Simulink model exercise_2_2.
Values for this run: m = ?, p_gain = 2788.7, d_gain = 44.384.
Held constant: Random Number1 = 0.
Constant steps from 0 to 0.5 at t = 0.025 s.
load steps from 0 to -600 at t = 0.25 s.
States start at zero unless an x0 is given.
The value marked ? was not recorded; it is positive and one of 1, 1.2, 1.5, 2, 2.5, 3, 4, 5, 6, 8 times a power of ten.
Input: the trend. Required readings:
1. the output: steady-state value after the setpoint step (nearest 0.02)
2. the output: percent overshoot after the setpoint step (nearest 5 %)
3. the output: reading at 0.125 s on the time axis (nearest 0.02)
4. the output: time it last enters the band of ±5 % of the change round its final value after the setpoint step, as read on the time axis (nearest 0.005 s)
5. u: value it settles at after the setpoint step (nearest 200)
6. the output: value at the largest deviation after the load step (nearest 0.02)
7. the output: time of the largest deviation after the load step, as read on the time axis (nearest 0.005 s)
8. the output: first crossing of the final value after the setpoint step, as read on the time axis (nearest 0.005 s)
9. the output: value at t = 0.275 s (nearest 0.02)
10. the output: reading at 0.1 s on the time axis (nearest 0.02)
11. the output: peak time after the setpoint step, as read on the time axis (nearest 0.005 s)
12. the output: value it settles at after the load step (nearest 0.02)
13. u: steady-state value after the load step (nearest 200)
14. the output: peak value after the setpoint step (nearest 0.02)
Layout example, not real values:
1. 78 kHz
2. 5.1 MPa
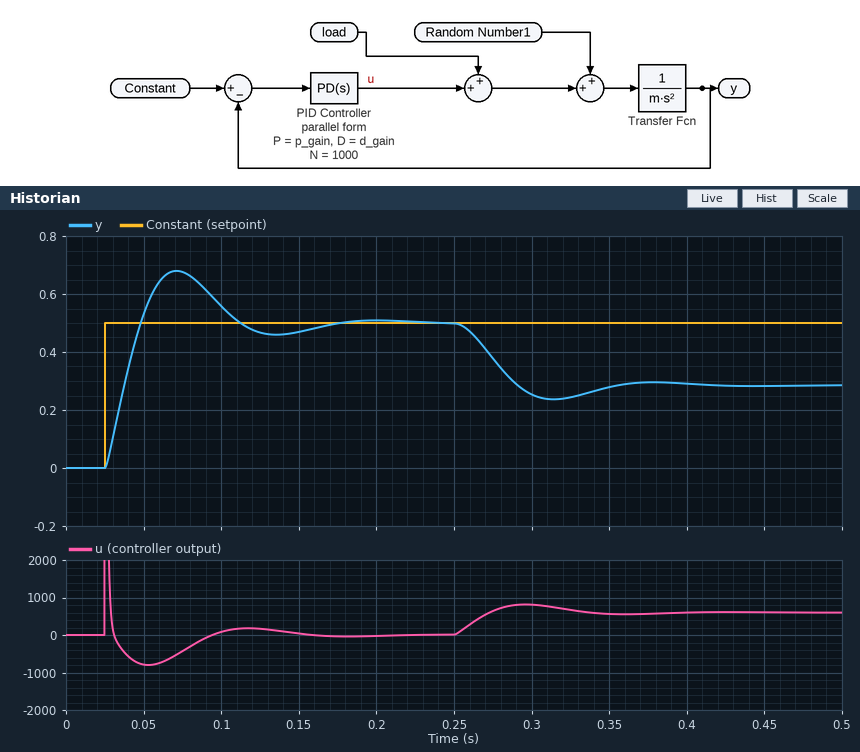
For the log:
1. 0.50
2. 35 %
3. 0.46
4. 0.155 s
5. 0
6. 0.24
7. 0.315 s
8. 0.050 s
9. 0.38
10. 0.56
11. 0.070 s
12. 0.28
13. 600
14. 0.68
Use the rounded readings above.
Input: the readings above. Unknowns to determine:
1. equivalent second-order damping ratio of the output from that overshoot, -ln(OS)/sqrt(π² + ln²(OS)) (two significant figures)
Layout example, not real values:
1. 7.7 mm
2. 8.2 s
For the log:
1. 0.32
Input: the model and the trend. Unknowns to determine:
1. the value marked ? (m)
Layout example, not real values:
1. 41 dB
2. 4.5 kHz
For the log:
1. 1
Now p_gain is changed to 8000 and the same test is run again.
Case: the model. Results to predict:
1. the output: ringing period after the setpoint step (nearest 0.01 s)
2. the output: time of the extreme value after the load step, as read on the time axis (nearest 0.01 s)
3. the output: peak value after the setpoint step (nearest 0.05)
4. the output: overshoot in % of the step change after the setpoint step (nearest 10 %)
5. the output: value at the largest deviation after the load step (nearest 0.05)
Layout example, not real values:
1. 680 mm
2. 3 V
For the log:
1. 0.07 s
2. 0.29 s
3. 0.75
4. 50 %
5. 0.40
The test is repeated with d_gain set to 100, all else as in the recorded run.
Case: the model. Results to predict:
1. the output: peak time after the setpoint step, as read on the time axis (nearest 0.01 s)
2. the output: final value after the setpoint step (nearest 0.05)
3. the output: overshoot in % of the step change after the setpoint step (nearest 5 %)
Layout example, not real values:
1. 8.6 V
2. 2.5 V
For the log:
1. 0.06 s
2. 0.50
3. 15 %
